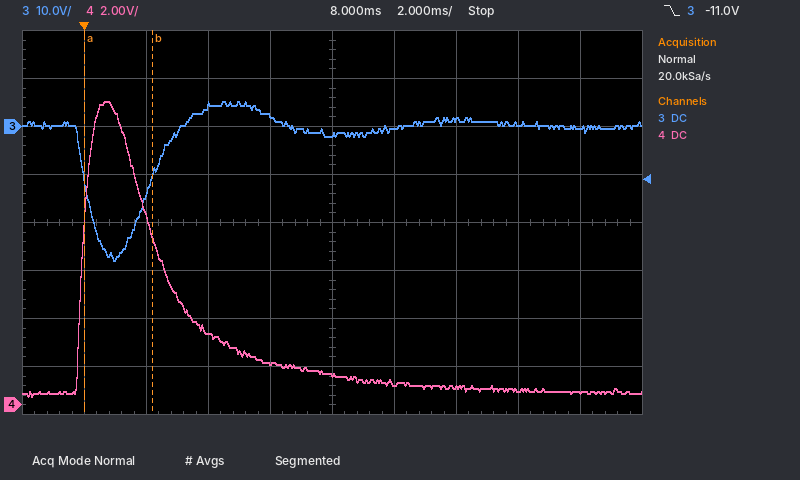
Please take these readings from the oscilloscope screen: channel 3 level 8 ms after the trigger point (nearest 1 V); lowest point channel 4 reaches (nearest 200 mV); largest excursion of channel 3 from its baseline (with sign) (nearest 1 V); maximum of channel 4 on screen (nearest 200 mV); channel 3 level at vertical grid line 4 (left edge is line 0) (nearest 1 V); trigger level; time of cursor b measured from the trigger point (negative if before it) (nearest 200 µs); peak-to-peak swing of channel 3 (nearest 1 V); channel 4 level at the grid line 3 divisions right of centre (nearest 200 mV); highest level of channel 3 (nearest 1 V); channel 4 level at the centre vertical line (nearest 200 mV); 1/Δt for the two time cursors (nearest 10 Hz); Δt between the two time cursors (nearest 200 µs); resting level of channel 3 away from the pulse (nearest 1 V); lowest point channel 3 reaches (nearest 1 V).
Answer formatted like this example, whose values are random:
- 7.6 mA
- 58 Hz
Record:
- -2 V
- 400 mV
- -28 V
- 12.6 V
- 2 V
- -11.0 V
- +2.2 ms
- 33 V
- 600 mV
- 5 V
- 1.2 V
- 450 Hz
- 2.2 ms
- 0 V
- -28 V
